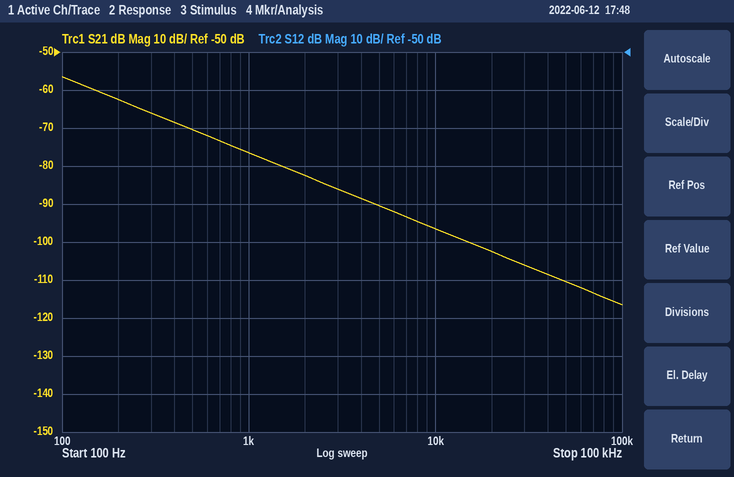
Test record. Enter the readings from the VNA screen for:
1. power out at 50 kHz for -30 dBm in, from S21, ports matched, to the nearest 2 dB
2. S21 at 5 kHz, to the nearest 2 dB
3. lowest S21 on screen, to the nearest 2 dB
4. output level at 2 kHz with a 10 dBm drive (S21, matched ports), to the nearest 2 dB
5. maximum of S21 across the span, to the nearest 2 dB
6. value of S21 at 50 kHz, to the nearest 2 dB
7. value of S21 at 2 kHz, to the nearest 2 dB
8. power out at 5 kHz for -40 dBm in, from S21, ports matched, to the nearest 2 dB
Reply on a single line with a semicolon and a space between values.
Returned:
-140 dBm; -90 dB; -116 dB; -72 dBm; -56 dB; -110 dB; -82 dB; -130 dBm
